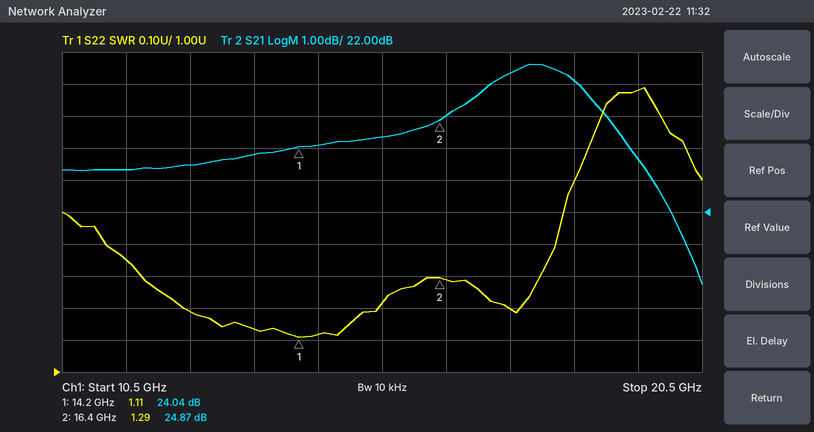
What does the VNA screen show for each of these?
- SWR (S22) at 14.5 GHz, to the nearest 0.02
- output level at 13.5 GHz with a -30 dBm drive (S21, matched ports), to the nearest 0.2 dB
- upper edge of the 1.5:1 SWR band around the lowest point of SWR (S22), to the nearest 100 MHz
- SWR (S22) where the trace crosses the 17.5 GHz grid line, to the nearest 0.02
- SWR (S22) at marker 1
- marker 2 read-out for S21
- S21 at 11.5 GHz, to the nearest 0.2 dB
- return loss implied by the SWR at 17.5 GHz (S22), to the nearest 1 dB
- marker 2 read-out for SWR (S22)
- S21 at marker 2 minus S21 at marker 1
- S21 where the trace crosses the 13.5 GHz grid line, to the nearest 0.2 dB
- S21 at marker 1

1.12
-6.2 dBm
18.3 GHz
1.20
1.11
24.87 dB
23.4 dB
21 dB
1.29
0.83 dB
23.8 dB
24.04 dB
